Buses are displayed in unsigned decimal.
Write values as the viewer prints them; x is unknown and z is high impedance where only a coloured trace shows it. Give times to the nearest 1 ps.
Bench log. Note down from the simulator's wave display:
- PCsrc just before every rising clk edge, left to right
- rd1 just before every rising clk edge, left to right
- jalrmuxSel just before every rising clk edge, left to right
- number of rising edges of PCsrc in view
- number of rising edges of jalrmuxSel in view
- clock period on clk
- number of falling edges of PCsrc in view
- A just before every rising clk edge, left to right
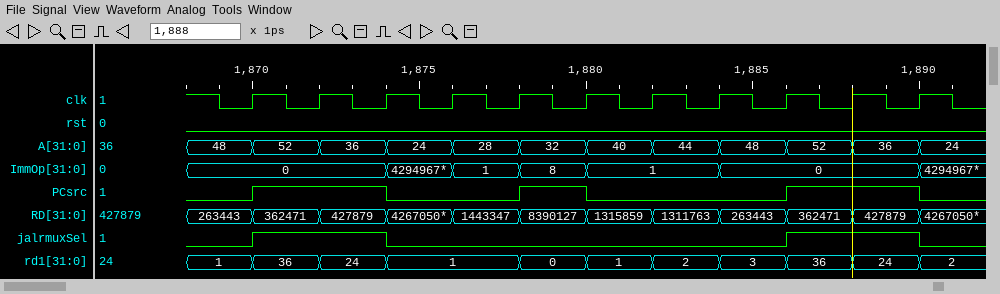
0 1 1 0 0 1 0 0 0 1 1
1, 36, 24, 1, 1, 0, 1, 2, 3, 36, 24
0 1 1 0 0 0 0 0 0 1 1
3
2
2 ps
3
48, 52, 36, 24, 28, 32, 40, 44, 48, 52, 36
